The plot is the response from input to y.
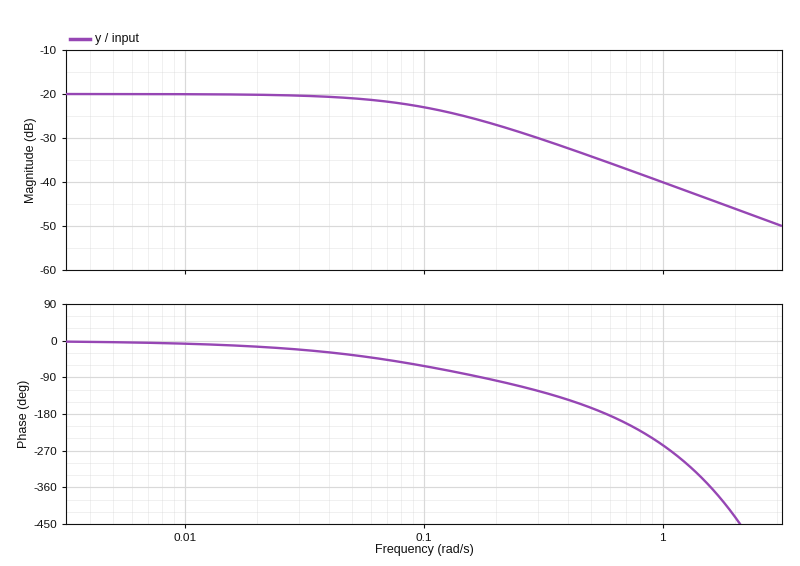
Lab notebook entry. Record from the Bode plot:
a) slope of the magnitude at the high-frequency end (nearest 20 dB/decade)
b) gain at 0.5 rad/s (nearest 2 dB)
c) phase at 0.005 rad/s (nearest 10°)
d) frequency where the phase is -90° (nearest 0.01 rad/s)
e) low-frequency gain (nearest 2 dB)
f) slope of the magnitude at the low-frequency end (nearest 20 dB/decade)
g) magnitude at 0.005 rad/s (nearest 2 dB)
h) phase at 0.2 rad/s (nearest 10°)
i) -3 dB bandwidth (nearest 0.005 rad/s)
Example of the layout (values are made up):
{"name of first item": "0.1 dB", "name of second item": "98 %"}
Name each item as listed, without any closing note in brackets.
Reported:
{"slope of the magnitude at the high-frequency end": "-20 dB/decade", "gain at 0.5 rad/s": "-34 dB", "phase at 0.005 rad/s": "0°", "frequency where the phase is -90°": "0.17 rad/s", "low-frequency gain": "-20 dB", "slope of the magnitude at the low-frequency end": "0 dB/decade", "magnitude at 0.005 rad/s": "-20 dB", "phase at 0.2 rad/s": "-100°", "-3 dB bandwidth": "0.100 rad/s"}
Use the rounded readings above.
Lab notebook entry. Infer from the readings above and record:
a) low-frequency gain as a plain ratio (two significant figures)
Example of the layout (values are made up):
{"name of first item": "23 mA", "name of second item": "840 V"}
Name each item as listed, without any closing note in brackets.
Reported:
{"low-frequency gain as a plain ratio": "0.10"}
